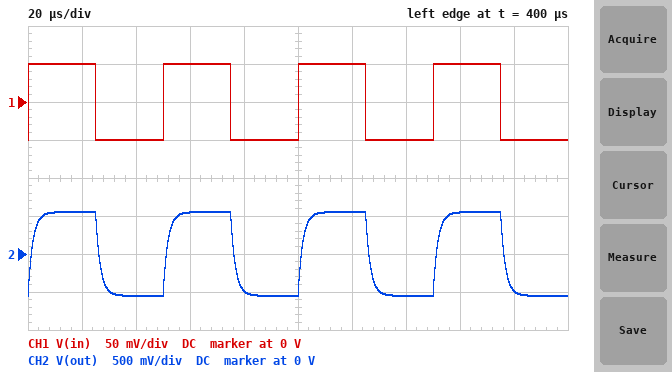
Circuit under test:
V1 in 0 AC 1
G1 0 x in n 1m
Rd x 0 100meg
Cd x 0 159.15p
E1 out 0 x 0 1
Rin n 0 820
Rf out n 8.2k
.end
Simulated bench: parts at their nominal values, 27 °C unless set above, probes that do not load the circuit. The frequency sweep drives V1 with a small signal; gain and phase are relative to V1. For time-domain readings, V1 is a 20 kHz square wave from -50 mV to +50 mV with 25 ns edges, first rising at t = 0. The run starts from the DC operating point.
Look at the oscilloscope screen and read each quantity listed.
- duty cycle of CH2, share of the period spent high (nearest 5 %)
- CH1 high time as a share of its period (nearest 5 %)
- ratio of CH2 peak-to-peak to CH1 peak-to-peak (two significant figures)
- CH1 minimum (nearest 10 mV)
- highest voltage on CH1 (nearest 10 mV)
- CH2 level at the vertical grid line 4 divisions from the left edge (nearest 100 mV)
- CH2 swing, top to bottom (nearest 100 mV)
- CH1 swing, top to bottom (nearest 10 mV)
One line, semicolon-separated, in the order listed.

50 %; 50 %; 11; -50 mV; 50 mV; -500 mV; 1.1 V; 100 mV
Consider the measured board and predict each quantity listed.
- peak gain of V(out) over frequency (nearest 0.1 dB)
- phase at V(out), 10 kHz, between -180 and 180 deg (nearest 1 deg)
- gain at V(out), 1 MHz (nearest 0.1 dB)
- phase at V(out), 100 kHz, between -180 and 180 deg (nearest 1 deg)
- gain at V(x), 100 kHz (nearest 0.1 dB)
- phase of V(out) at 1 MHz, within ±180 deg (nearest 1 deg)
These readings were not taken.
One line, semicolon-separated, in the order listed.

20.8 dB; -6 deg; 0 dB; -48 deg; 17.4 dB; -85 deg
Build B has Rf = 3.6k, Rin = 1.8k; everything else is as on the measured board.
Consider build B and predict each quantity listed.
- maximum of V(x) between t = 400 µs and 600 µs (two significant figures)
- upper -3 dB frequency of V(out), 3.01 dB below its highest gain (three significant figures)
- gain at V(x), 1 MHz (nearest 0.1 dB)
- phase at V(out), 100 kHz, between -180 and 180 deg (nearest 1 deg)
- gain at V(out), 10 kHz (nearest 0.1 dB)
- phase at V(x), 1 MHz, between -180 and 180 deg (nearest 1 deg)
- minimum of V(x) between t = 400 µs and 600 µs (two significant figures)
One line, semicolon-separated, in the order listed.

150 mV; 333 kHz; -0.5 dB; -17 deg; 9.5 dB; -72 deg; -150 mV
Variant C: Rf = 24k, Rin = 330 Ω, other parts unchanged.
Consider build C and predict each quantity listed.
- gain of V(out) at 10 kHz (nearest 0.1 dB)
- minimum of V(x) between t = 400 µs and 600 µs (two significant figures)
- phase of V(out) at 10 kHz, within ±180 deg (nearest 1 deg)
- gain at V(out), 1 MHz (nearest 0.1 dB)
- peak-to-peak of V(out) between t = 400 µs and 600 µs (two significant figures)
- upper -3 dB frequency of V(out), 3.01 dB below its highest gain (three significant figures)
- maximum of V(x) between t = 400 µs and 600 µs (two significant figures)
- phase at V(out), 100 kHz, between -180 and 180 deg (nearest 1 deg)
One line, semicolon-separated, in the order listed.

35.5 dB; -2.9 V; -36 deg; 0 dB; 5.8 V; 13.6 kHz; 2.9 V; -82 deg
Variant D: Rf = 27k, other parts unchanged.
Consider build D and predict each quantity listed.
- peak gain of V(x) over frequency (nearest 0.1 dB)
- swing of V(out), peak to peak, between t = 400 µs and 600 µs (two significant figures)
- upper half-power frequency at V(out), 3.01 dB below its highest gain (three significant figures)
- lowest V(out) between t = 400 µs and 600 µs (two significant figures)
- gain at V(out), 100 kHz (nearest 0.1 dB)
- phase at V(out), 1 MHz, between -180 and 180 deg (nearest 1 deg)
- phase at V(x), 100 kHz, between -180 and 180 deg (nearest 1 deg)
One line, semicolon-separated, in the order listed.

30.6 dB; 3.3 V; 29.5 kHz; -1.7 V; 19.6 dB; -88 deg; -74 deg
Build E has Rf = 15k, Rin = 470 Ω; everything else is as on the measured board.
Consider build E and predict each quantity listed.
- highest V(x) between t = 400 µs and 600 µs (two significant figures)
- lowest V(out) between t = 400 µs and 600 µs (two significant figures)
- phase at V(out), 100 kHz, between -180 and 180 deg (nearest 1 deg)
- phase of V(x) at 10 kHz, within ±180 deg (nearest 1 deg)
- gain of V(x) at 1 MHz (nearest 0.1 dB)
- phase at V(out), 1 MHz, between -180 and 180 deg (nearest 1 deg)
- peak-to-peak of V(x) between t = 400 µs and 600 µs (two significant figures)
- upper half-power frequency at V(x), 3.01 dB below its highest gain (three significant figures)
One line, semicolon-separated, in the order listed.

1.6 V; -1.6 V; -73 deg; -18 deg; 0 dB; -88 deg; 3.2 V; 30.4 kHz
